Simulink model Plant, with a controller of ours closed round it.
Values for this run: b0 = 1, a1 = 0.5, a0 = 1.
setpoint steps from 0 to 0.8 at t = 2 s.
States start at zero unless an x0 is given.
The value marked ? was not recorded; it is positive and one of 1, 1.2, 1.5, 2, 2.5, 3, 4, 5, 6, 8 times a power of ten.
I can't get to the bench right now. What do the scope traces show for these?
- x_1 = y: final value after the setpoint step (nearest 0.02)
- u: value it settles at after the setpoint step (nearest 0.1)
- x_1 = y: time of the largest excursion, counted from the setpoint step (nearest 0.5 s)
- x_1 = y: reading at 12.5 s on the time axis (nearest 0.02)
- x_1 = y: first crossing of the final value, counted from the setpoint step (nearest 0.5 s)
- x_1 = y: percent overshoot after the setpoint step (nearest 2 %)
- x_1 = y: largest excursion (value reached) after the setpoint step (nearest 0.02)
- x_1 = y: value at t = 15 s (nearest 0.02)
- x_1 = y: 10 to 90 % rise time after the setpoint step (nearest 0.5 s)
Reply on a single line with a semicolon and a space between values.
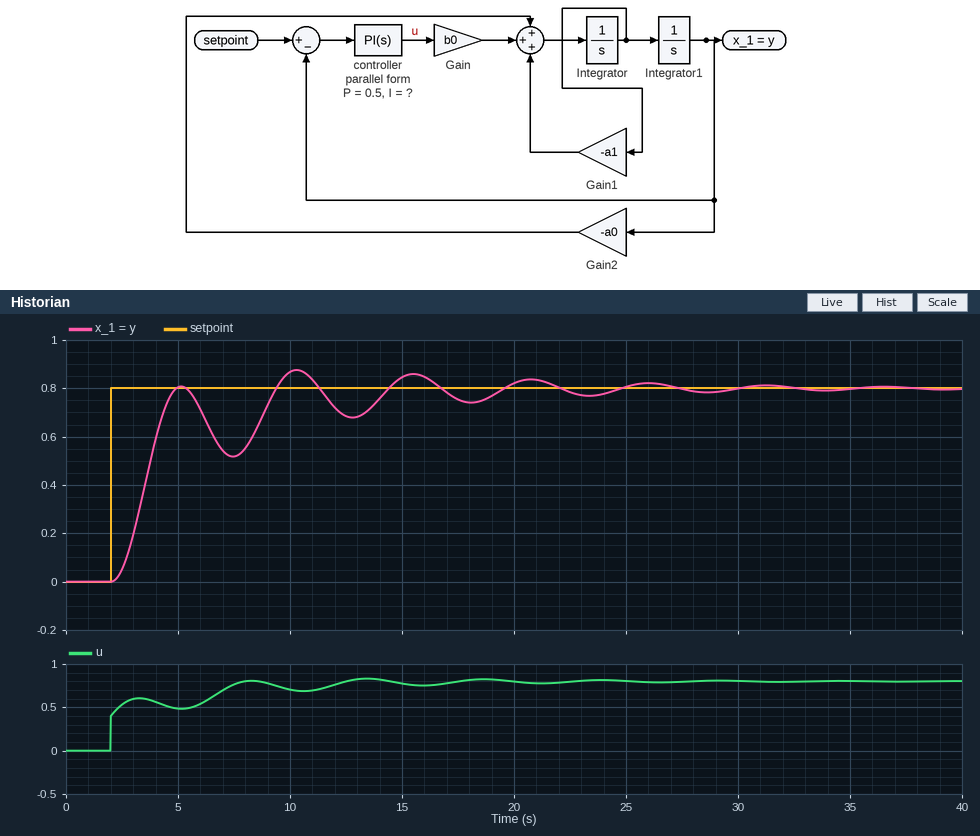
0.80; 0.8; 8.5 s; 0.68; 3.0 s; 10 %; 0.88; 0.84; 2.0 s
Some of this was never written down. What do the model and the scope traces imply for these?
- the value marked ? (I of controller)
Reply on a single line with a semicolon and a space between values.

0.4
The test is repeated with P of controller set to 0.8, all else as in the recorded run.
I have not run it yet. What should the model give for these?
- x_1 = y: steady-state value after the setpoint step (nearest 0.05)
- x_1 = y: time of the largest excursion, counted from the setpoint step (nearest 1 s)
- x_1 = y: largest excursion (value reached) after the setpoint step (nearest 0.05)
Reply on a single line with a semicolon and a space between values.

0.80; 7 s; 0.85
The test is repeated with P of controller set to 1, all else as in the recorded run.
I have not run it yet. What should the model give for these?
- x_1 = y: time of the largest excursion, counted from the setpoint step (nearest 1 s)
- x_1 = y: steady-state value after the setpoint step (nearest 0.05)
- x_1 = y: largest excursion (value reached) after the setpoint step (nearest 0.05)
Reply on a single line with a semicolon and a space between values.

7 s; 0.80; 0.85
